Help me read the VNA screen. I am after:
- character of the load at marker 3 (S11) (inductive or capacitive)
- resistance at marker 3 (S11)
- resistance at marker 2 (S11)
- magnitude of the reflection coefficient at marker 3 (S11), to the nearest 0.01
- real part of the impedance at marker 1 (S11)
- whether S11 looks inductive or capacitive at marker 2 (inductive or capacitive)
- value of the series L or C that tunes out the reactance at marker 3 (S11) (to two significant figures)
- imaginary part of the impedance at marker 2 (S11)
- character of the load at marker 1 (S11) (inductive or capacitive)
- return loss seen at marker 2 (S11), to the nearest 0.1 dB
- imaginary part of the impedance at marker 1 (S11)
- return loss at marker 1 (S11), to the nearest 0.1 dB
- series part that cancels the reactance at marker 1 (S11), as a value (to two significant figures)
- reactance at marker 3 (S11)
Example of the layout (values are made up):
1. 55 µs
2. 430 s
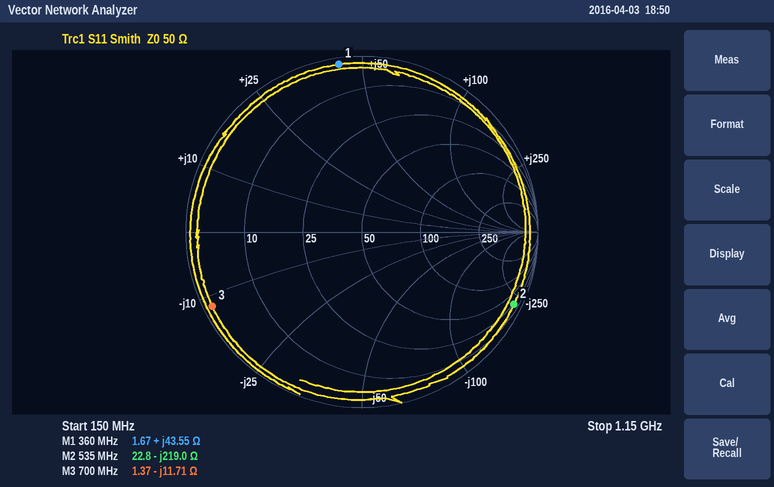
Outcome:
1. capacitive
2. 1.37 Ω
3. 22.8 Ω
4. 0.95
5. 1.67 Ω
6. capacitive
7. 2.7 nH
8. -219.0 Ω
9. inductive
10. 0.4 dB
11. +43.55 Ω
12. 0.3 dB
13. 10 pF
14. -11.71 Ω
